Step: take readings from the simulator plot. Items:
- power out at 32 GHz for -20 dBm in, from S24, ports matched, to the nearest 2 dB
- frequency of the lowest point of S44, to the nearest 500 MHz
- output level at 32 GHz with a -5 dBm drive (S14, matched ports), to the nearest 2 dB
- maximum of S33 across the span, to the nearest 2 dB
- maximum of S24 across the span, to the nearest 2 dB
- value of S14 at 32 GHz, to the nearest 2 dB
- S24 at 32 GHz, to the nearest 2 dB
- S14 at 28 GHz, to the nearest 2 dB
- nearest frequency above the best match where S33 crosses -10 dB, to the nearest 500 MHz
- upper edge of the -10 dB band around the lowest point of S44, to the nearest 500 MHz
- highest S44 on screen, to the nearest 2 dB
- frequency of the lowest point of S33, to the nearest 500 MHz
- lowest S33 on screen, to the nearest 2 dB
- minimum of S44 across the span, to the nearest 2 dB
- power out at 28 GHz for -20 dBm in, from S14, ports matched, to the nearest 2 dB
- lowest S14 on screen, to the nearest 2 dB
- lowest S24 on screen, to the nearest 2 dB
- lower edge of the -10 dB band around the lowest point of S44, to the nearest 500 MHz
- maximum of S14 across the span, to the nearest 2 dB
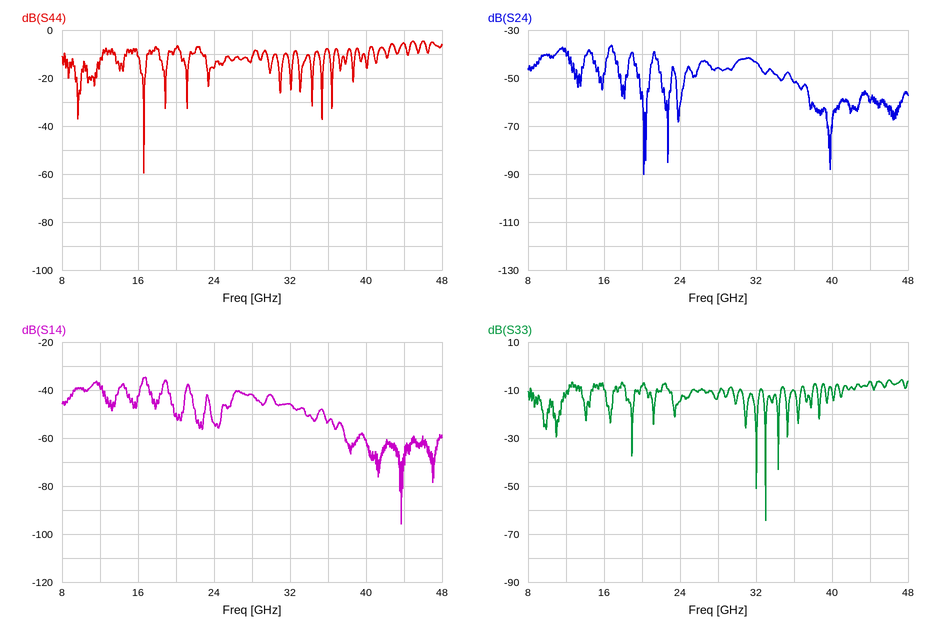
-64 dBm
16.5 GHz
-50 dBm
-6 dB
-36 dB
-46 dB
-44 dB
-42 dB
34.5 GHz
17.0 GHz
-4 dB
33.0 GHz
-64 dB
-60 dB
-62 dBm
-96 dB
-90 dB
16.0 GHz
-34 dB
